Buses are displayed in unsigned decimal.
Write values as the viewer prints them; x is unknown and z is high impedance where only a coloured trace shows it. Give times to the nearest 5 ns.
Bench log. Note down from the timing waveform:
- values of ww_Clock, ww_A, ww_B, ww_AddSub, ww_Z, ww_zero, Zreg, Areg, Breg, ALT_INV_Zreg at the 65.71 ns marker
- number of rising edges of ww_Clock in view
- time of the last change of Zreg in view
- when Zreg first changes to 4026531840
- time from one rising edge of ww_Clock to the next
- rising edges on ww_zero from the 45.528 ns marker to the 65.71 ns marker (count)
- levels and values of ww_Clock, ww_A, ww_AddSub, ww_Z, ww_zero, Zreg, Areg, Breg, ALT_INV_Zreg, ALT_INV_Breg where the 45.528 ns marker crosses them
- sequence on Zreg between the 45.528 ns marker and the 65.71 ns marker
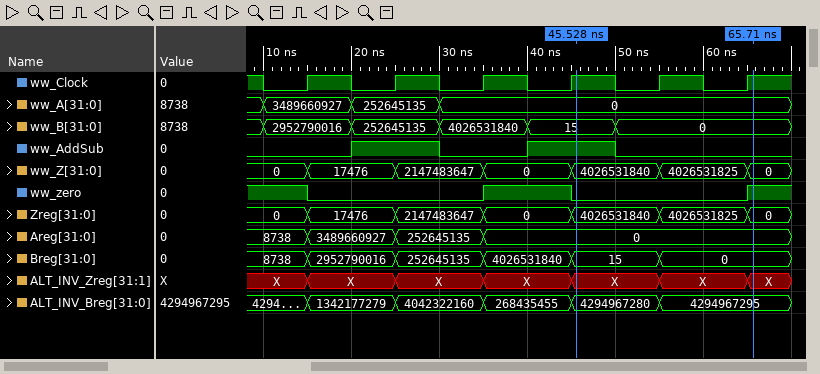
ww_Clock=1, ww_A=0, ww_B=0, ww_AddSub=0, ww_Z=0, ww_zero=1, Zreg=0, Areg=0, Breg=0, ALT_INV_Zreg=X
6
65 ns
45 ns
10 ns
1
ww_Clock=1, ww_A=0, ww_AddSub=1, ww_Z=4026531840, ww_zero=0, Zreg=4026531840, Areg=0, Breg=15, ALT_INV_Zreg=X, ALT_INV_Breg=4294967280
4026531840, 4026531825, 0
